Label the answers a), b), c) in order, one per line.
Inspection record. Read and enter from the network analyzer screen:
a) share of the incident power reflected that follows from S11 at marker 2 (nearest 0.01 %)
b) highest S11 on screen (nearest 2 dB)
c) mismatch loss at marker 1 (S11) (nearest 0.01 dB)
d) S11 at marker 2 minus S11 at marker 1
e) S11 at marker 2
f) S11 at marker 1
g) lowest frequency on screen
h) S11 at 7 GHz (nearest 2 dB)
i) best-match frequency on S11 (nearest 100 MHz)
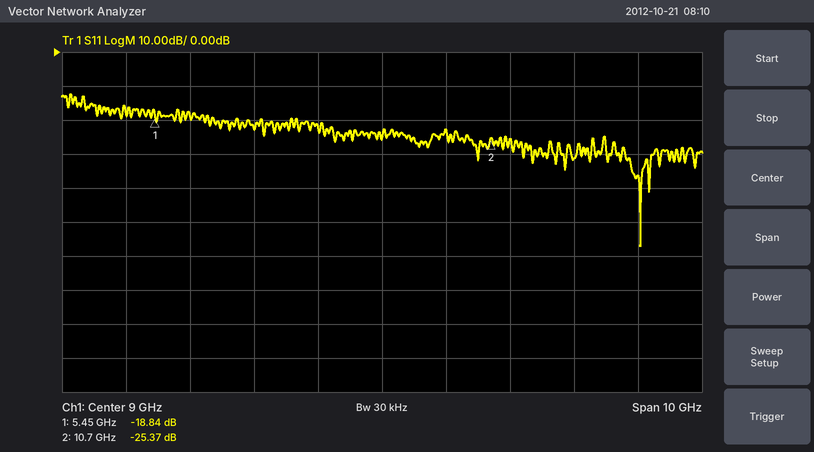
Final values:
a) 0.29 %
b) -12 dB
c) 0.06 dB
d) -6.53 dB
e) -25.37 dB
f) -18.84 dB
g) 4 GHz
h) -22 dB
i) 13.0 GHz
